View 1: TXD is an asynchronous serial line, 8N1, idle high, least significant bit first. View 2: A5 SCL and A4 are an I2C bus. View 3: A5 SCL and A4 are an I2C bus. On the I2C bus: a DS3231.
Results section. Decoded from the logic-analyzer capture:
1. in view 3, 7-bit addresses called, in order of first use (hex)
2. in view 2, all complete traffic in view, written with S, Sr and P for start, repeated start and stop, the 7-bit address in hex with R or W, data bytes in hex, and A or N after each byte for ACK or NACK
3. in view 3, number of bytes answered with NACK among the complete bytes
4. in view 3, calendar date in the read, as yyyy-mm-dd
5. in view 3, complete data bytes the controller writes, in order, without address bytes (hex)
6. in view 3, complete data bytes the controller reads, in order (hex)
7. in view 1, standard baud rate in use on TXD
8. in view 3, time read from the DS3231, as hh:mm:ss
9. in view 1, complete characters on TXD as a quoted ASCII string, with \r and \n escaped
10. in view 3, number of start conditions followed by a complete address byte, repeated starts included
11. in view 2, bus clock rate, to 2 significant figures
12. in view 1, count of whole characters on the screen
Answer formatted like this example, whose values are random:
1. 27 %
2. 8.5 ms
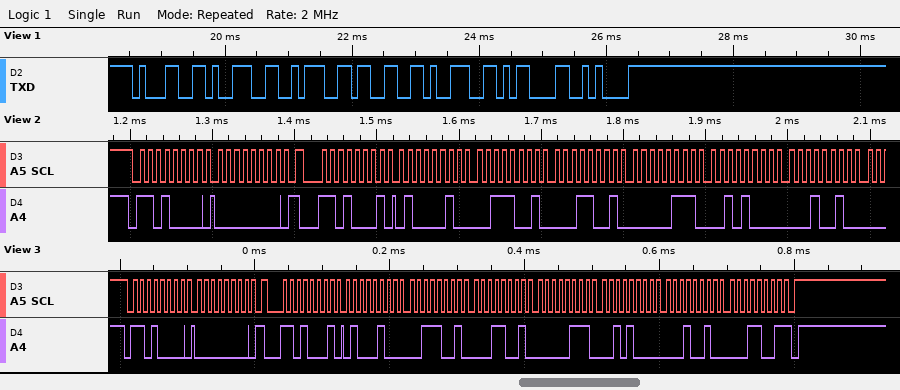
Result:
1. 0x68
2. S 68W A 00 A Sr 68R A 42 A 39 A 19 A 07 A 28 A 12 A
3. 1
4. 2019-12-28
5. 00
6. 44 39 19 07 28 12 19
7. 9600 baud
8. 19:39:44
9. "19:39\r\n"
10. 2
11. 100 kHz
12. 7
